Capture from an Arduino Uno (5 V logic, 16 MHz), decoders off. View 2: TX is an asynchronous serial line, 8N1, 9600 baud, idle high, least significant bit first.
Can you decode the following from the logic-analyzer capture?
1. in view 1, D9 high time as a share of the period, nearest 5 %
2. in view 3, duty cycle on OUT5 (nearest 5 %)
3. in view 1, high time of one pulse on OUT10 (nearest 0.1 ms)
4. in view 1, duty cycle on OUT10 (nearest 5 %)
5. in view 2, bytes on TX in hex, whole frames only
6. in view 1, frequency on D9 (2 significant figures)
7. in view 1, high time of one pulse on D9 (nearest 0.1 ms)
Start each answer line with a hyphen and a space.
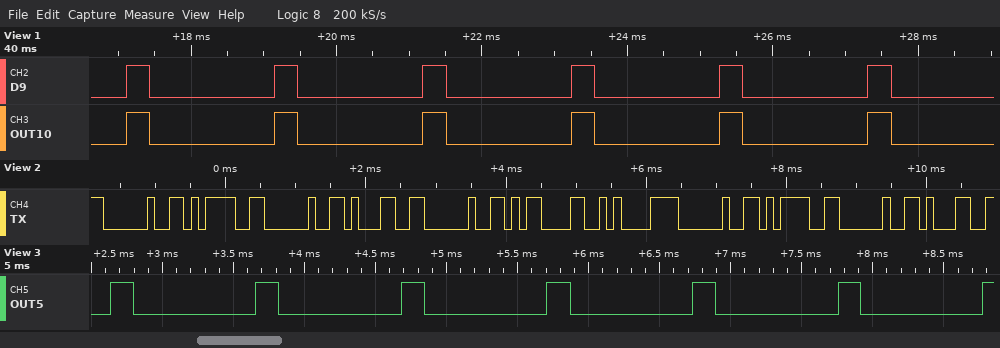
- 15 %
- 15 %
- 0.3 ms
- 15 %
- 20 3D 20 31 20 0D 0A 20 3D 20 31
- 490 Hz
- 0.3 ms
